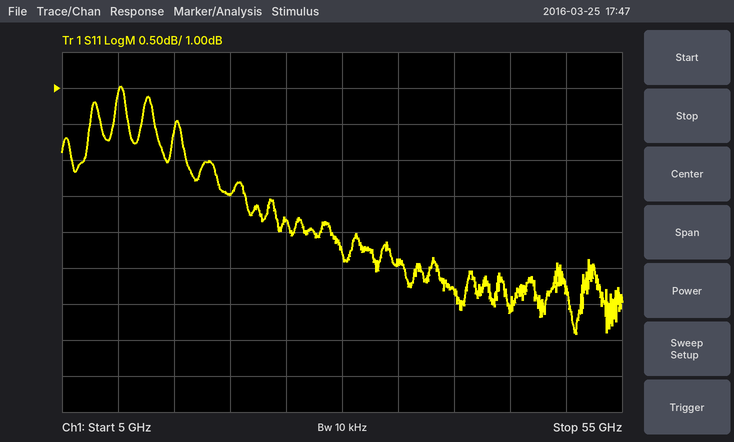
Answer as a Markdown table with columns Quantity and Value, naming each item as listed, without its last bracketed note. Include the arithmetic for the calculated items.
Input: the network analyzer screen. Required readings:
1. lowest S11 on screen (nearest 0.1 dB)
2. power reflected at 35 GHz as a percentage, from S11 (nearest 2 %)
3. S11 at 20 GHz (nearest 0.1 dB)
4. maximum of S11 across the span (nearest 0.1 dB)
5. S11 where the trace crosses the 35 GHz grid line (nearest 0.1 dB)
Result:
| Quantity | Value |
|---|---|
| lowest S11 on screen | -2.4 dB |
| power reflected at 35 GHz as a percentage, from S11 | 10^(-1.4/10) ≈ 72 % |
| S11 at 20 GHz | -0.5 dB |
| maximum of S11 across the span | 1.0 dB |
| S11 where the trace crosses the 35 GHz grid line | -1.4 dB |
